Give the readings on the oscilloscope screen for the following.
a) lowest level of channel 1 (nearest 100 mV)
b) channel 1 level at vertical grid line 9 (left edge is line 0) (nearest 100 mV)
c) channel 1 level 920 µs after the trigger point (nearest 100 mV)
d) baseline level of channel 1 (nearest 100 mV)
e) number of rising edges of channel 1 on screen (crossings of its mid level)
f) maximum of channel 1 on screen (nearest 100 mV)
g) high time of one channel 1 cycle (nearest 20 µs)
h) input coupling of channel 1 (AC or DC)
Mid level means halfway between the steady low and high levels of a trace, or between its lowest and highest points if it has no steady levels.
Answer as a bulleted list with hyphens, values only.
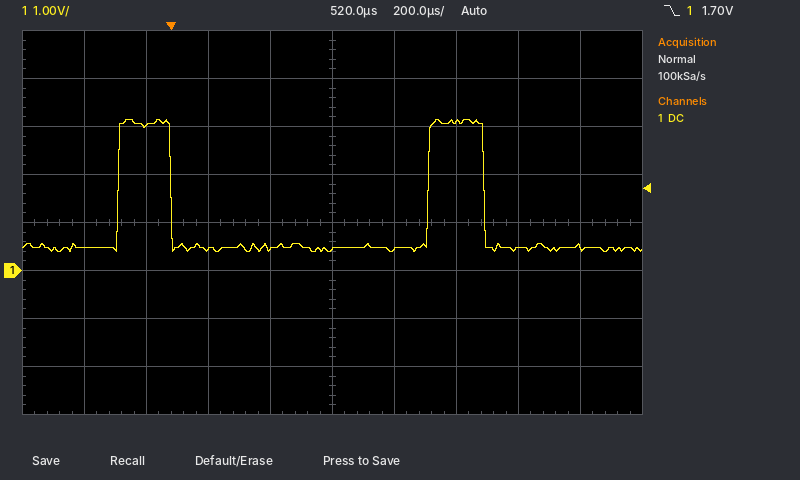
- 400 mV
- 500 mV
- 3.1 V
- 500 mV
- 2
- 3.1 V
- 180 µs
- DC
